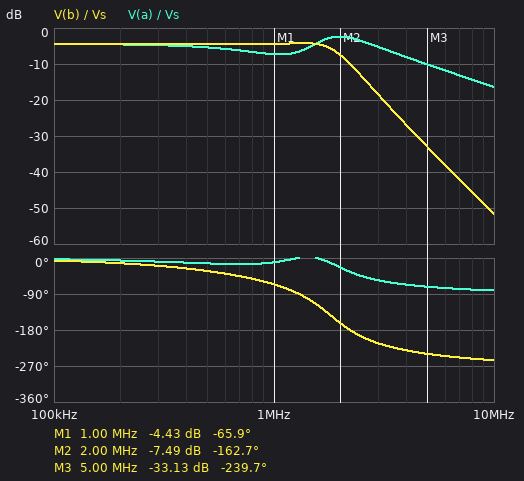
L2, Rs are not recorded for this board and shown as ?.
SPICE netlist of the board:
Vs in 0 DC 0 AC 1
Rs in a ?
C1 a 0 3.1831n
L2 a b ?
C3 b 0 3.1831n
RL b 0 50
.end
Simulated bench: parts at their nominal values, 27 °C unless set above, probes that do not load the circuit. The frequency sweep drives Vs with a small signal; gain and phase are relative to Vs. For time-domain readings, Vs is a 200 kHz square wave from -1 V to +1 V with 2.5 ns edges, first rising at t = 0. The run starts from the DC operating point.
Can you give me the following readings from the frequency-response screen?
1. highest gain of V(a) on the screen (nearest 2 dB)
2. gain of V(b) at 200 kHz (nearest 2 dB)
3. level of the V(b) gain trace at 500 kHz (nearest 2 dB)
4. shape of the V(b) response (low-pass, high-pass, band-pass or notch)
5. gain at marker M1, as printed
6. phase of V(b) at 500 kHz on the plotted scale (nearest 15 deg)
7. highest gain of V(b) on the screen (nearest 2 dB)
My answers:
-2 dB
-4 dB
-4 dB
low-pass
-4.43 dB
-30 deg
-4 dB
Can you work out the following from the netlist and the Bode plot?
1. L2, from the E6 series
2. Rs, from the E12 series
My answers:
4.7 µH
33 Ω
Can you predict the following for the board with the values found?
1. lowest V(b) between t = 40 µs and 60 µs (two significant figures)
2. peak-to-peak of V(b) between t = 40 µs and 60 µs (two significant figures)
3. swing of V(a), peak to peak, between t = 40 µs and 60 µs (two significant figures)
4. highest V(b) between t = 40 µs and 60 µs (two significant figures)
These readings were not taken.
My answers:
-740 mV
1.5 V
1.3 V
740 mV
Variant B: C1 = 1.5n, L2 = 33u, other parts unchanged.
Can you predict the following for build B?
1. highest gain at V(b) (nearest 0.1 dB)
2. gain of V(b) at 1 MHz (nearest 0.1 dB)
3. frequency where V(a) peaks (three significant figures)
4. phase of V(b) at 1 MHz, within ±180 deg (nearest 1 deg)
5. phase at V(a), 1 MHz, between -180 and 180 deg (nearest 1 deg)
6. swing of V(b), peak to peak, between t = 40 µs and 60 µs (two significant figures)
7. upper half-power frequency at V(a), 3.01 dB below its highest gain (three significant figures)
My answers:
-4.4 dB
-14.6 dB
1.03 MHz
-135 deg
-7 deg
1.2 V
3.57 MHz
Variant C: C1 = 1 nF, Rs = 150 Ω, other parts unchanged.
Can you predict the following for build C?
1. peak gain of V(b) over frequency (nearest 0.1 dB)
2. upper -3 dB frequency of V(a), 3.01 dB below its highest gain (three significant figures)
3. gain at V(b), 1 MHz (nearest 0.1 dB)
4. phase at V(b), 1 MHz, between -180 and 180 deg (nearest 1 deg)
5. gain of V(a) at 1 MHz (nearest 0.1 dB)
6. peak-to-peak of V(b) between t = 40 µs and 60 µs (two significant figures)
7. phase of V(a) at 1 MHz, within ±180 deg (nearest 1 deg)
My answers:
-12.0 dB
3.33 MHz
-13.8 dB
-54 deg
-16.7 dB
530 mV
1 deg
